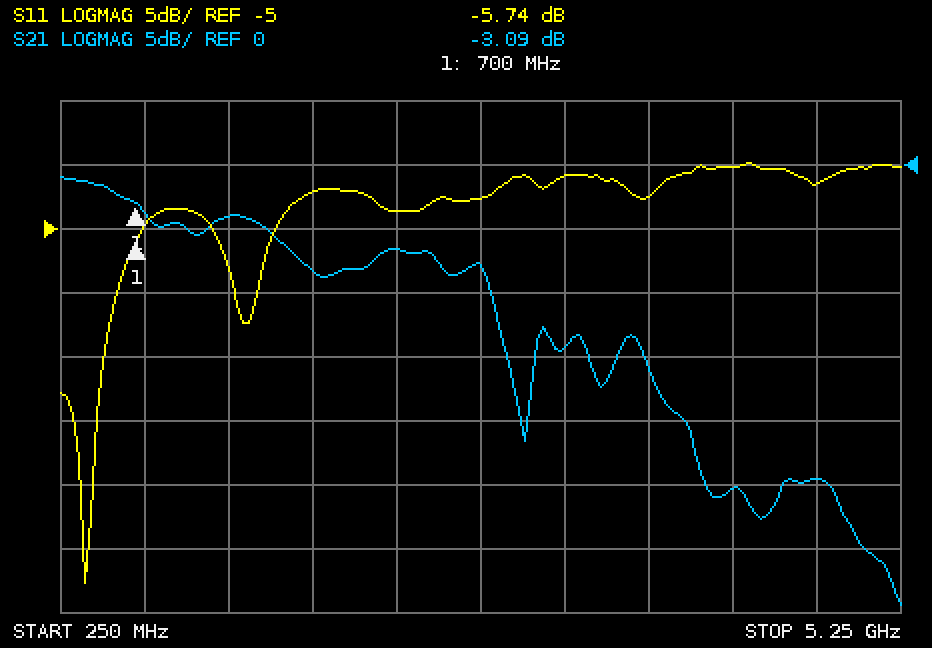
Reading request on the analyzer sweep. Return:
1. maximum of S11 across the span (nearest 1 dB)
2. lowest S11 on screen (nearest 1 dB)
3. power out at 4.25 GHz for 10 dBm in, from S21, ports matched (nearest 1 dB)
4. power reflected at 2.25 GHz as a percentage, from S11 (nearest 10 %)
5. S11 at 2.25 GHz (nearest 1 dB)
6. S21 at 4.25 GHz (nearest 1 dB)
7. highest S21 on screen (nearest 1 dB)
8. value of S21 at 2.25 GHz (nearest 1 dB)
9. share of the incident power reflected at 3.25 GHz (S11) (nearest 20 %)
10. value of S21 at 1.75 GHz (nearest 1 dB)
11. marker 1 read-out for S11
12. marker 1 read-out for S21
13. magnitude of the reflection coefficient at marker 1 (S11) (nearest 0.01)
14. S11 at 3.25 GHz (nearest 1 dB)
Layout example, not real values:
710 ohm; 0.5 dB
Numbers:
0 dB; -33 dB; -15 dBm; 40 %; -4 dB; -25 dB; -1 dB; -7 dB; 80 %; -8 dB; -5.74 dB; -3.09 dB; 0.52; -1 dB
